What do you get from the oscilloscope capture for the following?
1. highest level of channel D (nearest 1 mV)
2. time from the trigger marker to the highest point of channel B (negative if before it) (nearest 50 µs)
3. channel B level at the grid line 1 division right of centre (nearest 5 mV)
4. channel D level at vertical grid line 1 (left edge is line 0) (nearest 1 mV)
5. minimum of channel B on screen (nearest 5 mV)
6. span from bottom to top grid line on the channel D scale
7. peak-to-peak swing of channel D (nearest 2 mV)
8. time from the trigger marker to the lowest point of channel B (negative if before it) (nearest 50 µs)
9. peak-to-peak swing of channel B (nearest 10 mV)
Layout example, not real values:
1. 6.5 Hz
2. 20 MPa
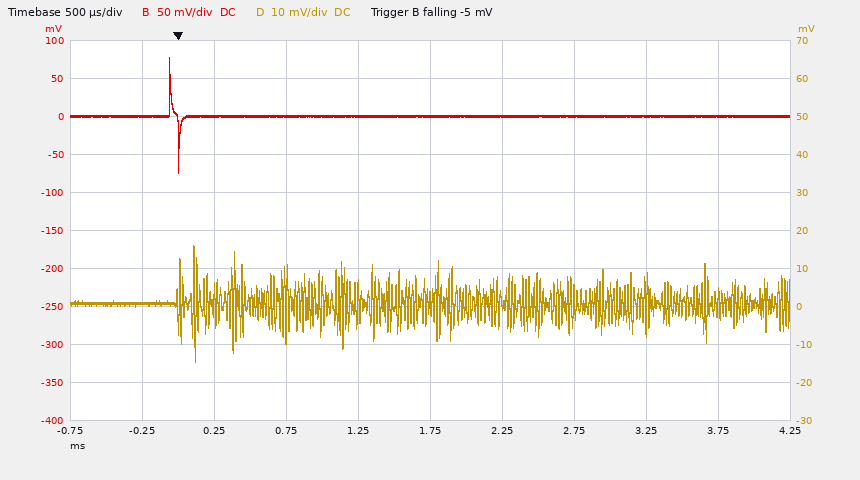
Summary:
1. 16 mV
2. -50 µs
3. 0 mV
4. 1 mV
5. -75 mV
6. 100 mV
7. 30 mV
8. 0 µs
9. 150 mV
